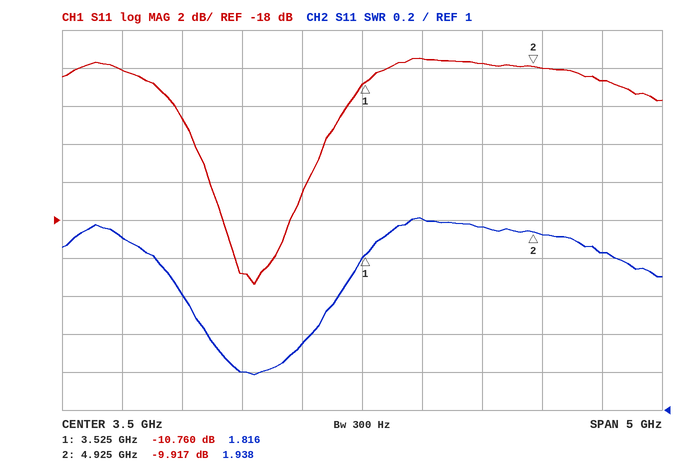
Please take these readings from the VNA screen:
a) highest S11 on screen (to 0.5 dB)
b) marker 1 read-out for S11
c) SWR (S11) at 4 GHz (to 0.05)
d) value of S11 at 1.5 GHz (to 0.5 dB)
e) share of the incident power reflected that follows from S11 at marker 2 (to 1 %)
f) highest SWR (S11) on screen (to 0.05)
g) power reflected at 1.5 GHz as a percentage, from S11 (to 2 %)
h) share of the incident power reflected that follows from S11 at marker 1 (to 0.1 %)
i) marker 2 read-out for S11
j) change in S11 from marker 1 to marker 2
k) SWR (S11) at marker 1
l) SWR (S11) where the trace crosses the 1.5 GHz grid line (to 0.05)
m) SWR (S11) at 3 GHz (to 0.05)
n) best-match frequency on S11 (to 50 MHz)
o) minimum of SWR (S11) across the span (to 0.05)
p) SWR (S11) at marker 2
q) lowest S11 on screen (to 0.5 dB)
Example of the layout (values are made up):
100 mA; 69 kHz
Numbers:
-9.5 dB; -10.760 dB; 2.00; -10.0 dB; 10 %; 2.00; 10 %; 8.4 %; -9.917 dB; 0.843 dB; 1.816; 1.90; 1.35; 2.60 GHz; 1.20; 1.938; -21.5 dB
